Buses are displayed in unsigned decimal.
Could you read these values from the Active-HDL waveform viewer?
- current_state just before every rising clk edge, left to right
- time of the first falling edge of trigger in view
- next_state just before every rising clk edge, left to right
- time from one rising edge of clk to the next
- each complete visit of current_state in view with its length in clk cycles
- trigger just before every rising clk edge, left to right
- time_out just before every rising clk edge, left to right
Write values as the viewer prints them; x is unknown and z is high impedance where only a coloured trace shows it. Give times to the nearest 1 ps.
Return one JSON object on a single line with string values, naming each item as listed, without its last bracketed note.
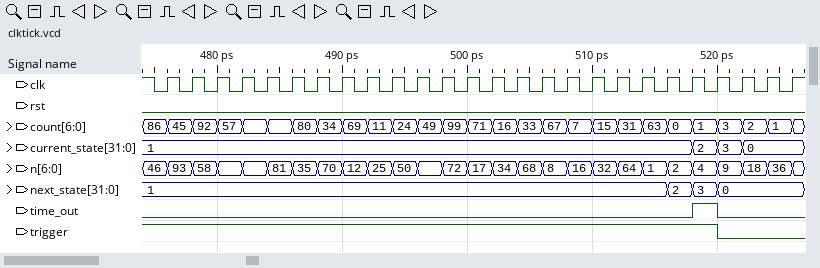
{"current_state just before every rising clk edge, left to right": "1, 1, 1, 1, 1, 1, 1, 1, 1, 1, 1, 1, 1, 1, 1, 1, 1, 1, 1, 1, 1, 1, 2, 3, 0, 0", "time of the first falling edge of trigger in view": "520 ps", "next_state just before every rising clk edge, left to right": "1, 1, 1, 1, 1, 1, 1, 1, 1, 1, 1, 1, 1, 1, 1, 1, 1, 1, 1, 1, 1, 2, 3, 0, 0, 0", "time from one rising edge of clk to the next": "2 ps", "each complete visit of current_state in view with its length in clk cycles": "2: 1, 3: 1", "trigger just before every rising clk edge, left to right": "1 1 1 1 1 1 1 1 1 1 1 1 1 1 1 1 1 1 1 1 1 1 1 0 0 0", "time_out just before every rising clk edge, left to right": "0 0 0 0 0 0 0 0 0 0 0 0 0 0 0 0 0 0 0 0 0 0 1 0 0 0"}
